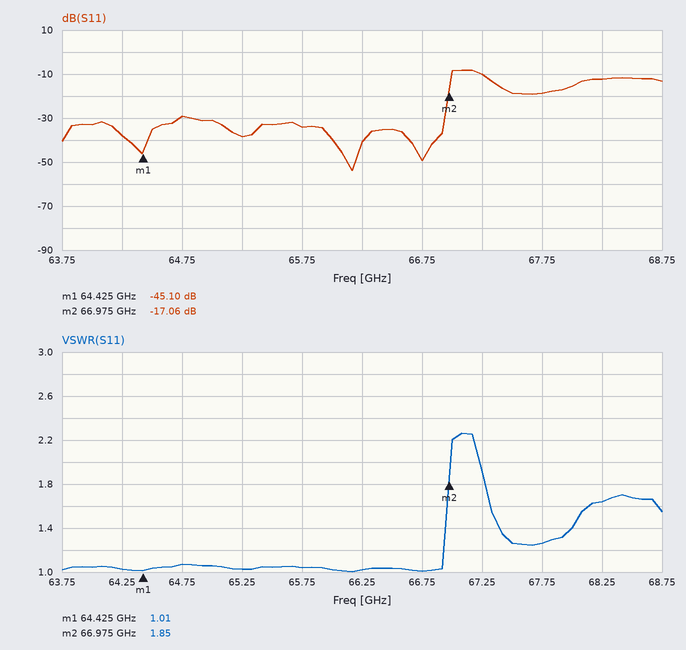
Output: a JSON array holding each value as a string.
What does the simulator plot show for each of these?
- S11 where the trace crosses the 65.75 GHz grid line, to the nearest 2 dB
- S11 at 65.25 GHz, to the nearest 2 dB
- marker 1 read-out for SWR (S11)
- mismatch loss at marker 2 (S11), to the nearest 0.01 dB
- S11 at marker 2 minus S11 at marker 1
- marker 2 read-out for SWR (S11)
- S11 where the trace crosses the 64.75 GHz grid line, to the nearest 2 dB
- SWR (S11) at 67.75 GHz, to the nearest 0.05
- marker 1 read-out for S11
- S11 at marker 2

["-34 dB", "-38 dB", "1.01", "0.09 dB", "28.04 dB", "1.85", "-30 dB", "1.25", "-45.10 dB", "-17.06 dB"]
